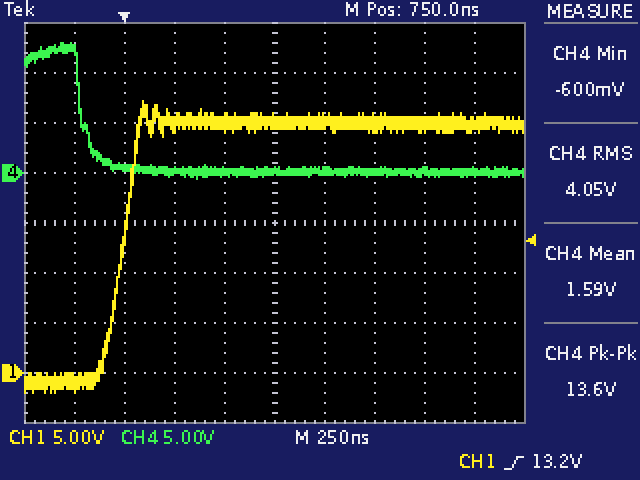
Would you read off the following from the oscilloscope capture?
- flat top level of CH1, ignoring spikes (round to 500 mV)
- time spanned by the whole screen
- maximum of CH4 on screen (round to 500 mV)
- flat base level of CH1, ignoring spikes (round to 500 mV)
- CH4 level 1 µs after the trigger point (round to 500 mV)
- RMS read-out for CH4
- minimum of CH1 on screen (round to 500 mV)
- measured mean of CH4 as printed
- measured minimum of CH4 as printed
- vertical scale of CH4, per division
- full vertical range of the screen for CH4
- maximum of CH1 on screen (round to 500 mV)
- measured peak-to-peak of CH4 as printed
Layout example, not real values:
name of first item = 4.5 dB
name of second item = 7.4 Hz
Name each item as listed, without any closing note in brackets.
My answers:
flat top level of CH1, ignoring spikes = 25.0 V
time spanned by the whole screen = 2.5 µs
maximum of CH4 on screen = 13.0 V
flat base level of CH1, ignoring spikes = -1.0 V
CH4 level 1 µs after the trigger point = 0.0 V
RMS read-out for CH4 = 4.05 V
minimum of CH1 on screen = -2.0 V
measured mean of CH4 as printed = 1.59 V
measured minimum of CH4 as printed = -600 mV
vertical scale of CH4, per division = 5 V
full vertical range of the screen for CH4 = 40 V
maximum of CH1 on screen = 27.0 V
measured peak-to-peak of CH4 as printed = 13.6 V
